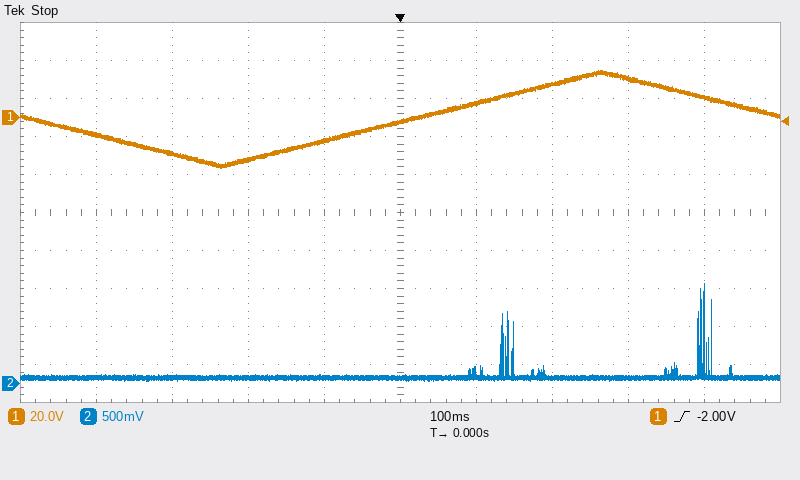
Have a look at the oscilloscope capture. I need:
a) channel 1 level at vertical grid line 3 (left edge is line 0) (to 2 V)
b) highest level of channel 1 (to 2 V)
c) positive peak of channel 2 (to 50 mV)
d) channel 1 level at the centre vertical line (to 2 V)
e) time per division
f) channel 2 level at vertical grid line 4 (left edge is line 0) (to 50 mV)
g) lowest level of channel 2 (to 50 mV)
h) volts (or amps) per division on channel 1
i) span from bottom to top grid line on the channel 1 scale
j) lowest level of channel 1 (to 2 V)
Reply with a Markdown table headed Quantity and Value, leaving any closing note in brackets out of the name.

| Quantity | Value |
|---|---|
| channel 1 level at vertical grid line 3 (left edge is line 0) | -22 V |
| highest level of channel 1 | 24 V |
| positive peak of channel 2 | 1.30 V |
| channel 1 level at the centre vertical line | -2 V |
| time per division | 100 ms |
| channel 2 level at vertical grid line 4 (left edge is line 0) | 100 mV |
| lowest level of channel 2 | 50 mV |
| volts (or amps) per division on channel 1 | 20 V |
| span from bottom to top grid line on the channel 1 scale | 200 V |
| lowest level of channel 1 | -26 V |
